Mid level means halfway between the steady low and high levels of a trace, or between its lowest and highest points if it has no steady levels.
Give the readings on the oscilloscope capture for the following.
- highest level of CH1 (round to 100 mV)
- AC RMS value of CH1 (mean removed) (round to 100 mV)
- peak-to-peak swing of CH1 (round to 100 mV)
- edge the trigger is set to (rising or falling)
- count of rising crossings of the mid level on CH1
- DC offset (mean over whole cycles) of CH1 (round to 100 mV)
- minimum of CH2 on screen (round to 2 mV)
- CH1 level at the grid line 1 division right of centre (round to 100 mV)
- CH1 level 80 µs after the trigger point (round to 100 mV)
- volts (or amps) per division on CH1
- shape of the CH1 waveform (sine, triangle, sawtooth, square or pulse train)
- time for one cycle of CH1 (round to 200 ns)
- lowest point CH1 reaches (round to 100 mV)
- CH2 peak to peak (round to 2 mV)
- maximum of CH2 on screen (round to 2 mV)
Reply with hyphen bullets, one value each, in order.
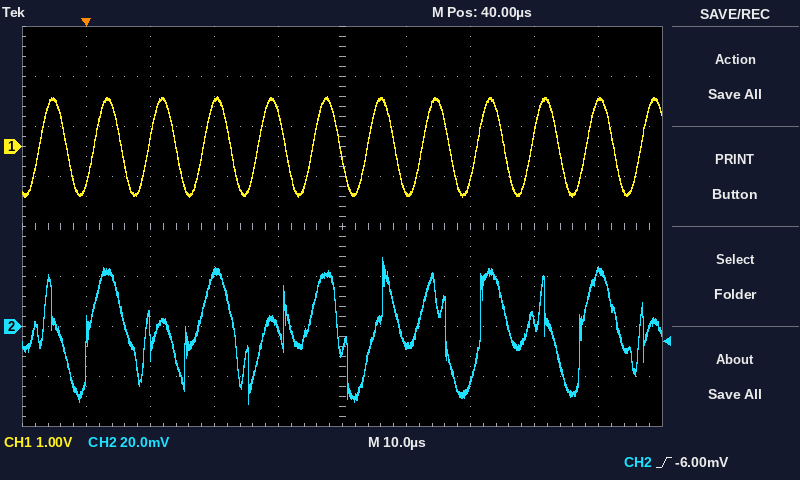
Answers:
- 1.0 V
- 700 mV
- 2.0 V
- rising
- 12
- 0.0 V
- -30 mV
- -900 mV
- 900 mV
- 1 V
- sine
- 8.6 µs
- -1.0 V
- 58 mV
- 28 mV
